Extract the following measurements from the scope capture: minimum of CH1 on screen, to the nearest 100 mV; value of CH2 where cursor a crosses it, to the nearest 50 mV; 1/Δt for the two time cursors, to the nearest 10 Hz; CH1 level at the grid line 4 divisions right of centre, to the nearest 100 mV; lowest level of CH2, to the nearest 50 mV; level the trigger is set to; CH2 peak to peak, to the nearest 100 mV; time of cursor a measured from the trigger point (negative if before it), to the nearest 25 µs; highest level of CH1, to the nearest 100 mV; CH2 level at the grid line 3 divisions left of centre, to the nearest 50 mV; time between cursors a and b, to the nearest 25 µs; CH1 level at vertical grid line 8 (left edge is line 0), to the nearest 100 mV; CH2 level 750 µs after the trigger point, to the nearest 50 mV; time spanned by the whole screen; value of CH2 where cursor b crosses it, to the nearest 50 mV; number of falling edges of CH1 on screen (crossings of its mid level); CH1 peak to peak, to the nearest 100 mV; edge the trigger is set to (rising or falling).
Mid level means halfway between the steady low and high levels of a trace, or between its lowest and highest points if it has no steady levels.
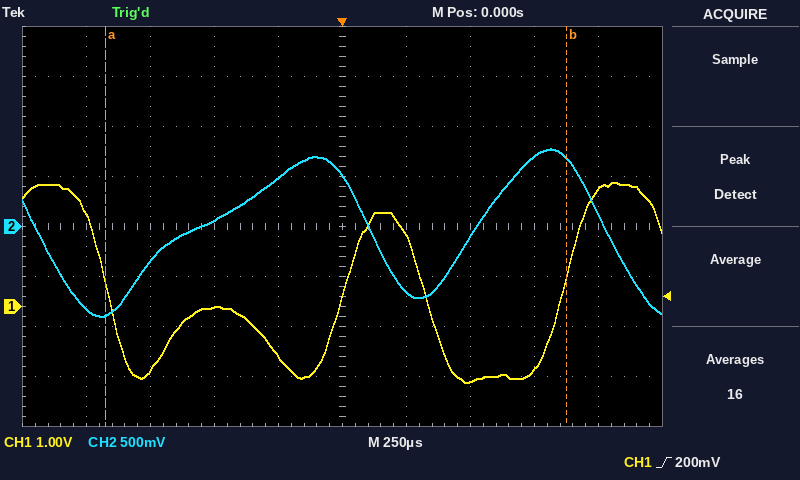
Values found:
-1.5 V
-900 mV
560 Hz
2.3 V
-900 mV
200 mV
1.70 V
-925 µs
2.5 V
-350 mV
1.800 ms
-1.3 V
700 mV
2.5 ms
700 mV
2
4.0 V
rising
